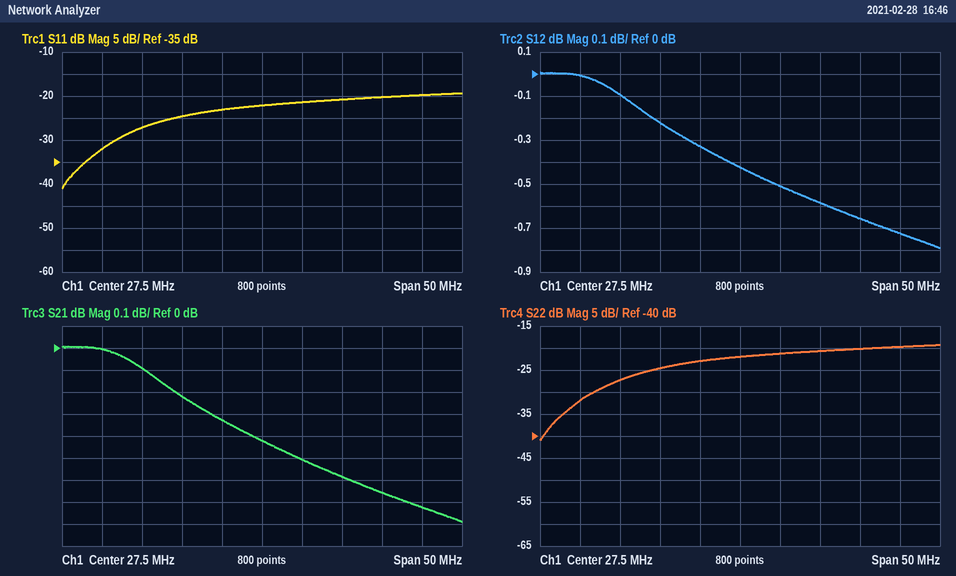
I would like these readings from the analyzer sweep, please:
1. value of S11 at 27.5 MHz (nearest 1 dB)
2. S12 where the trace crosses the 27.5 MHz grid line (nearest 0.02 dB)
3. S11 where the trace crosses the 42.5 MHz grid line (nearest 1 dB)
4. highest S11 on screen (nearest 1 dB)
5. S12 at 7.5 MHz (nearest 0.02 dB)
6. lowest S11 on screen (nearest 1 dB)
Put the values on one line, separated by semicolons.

-22 dB; -0.42 dB; -20 dB; -19 dB; 0.00 dB; -41 dB
